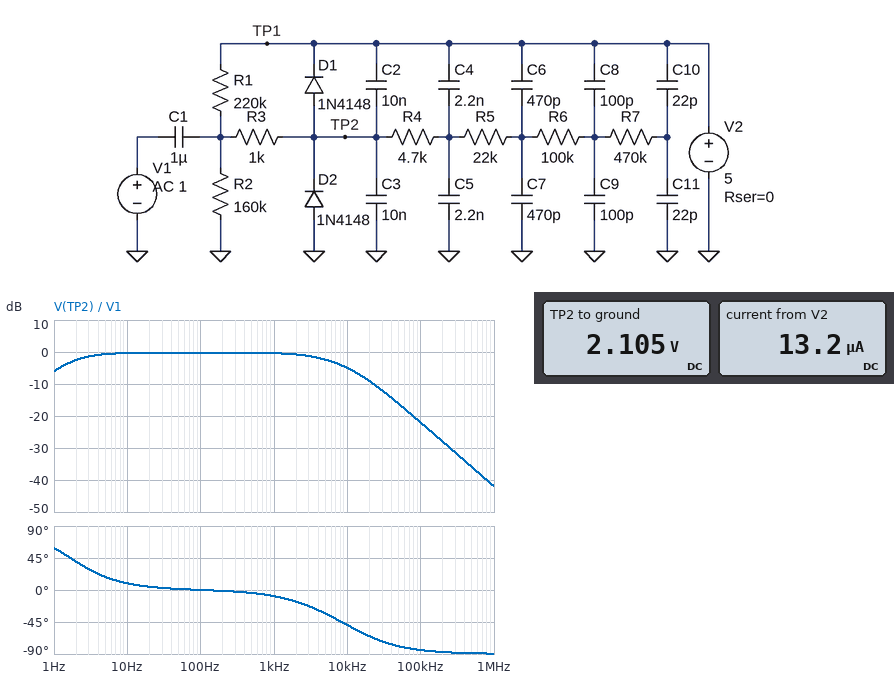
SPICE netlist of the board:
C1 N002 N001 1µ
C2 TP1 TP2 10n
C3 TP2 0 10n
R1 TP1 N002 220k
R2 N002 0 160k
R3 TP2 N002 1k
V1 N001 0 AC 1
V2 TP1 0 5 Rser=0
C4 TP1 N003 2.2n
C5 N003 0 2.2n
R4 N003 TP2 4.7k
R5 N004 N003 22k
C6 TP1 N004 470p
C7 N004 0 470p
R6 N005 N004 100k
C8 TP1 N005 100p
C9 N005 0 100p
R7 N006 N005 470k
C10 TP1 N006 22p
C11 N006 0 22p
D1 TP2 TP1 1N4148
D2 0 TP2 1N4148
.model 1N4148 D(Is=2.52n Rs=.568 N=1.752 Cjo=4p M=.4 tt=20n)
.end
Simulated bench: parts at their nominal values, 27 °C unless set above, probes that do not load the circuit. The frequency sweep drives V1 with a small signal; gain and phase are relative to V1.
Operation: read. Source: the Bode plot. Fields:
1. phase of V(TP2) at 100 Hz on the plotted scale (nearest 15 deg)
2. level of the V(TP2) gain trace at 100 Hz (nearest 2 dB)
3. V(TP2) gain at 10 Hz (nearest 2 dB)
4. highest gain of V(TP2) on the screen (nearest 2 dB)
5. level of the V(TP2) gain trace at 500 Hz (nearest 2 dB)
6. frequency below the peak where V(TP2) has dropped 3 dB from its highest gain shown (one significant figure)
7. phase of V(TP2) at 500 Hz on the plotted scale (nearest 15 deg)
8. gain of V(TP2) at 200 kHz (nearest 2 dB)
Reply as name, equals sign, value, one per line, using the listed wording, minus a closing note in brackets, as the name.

phase of V(TP2) at 100 Hz on the plotted scale = 0 deg
level of the V(TP2) gain trace at 100 Hz = 0 dB
V(TP2) gain at 10 Hz = 0 dB
highest gain of V(TP2) on the screen = 0 dB
level of the V(TP2) gain trace at 500 Hz = 0 dB
frequency below the peak where V(TP2) has dropped 3 dB from its highest gain shown = 2 Hz
phase of V(TP2) at 500 Hz on the plotted scale = 0 deg
gain of V(TP2) at 200 kHz = -28 dB
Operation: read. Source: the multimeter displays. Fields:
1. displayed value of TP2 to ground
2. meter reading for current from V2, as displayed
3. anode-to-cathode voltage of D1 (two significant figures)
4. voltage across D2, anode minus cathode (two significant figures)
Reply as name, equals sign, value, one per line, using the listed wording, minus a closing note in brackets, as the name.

displayed value of TP2 to ground = 2.105 V
meter reading for current from V2, as displayed = 13.2 µA
anode-to-cathode voltage of D1 = -2.9 V
voltage across D2, anode minus cathode = -2.1 V
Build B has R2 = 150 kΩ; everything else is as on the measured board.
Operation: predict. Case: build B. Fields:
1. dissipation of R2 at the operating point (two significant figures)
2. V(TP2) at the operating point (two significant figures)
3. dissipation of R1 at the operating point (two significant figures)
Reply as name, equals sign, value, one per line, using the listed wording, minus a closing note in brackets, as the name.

dissipation of R2 at the operating point = 27 µW
V(TP2) at the operating point = 2.0 V
dissipation of R1 at the operating point = 40 µW
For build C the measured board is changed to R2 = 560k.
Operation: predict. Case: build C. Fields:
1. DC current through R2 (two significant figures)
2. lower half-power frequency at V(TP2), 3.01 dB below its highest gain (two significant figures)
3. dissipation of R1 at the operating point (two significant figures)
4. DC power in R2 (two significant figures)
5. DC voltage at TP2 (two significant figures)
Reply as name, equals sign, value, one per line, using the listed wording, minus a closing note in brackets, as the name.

DC current through R2 = 6.4 µA
lower half-power frequency at V(TP2), 3.01 dB below its highest gain = 980 mHz
dissipation of R1 at the operating point = 9.0 µW
DC power in R2 = 23 µW
DC voltage at TP2 = 3.6 V
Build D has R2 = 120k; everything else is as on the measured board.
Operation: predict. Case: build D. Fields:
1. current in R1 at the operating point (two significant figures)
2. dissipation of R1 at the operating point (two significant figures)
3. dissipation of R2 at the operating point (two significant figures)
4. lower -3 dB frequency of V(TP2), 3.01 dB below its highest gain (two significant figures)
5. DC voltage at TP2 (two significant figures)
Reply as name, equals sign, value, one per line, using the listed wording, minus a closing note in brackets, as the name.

current in R1 at the operating point = 15 µA
dissipation of R1 at the operating point = 48 µW
dissipation of R2 at the operating point = 26 µW
lower -3 dB frequency of V(TP2), 3.01 dB below its highest gain = 2.0 Hz
DC voltage at TP2 = 1.8 V
